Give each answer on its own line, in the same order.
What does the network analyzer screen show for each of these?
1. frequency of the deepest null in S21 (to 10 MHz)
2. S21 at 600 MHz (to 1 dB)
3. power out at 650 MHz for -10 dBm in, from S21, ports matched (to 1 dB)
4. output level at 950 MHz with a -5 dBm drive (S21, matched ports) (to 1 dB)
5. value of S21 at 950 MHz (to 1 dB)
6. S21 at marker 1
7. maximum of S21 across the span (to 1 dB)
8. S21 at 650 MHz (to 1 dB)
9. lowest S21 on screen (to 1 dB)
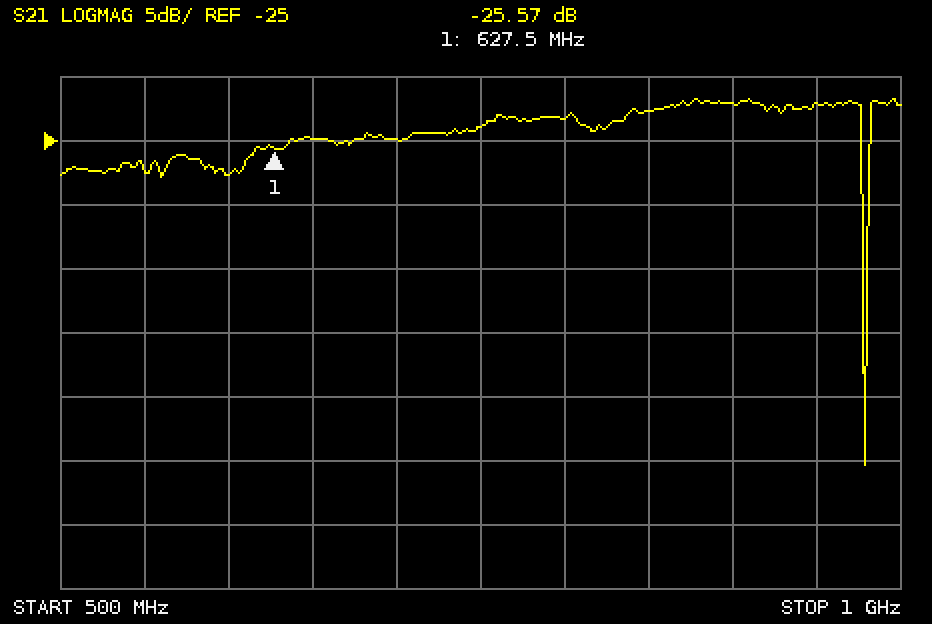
980 MHz
-28 dB
-35 dBm
-27 dBm
-22 dB
-25.57 dB
-22 dB
-25 dB
-50 dB
